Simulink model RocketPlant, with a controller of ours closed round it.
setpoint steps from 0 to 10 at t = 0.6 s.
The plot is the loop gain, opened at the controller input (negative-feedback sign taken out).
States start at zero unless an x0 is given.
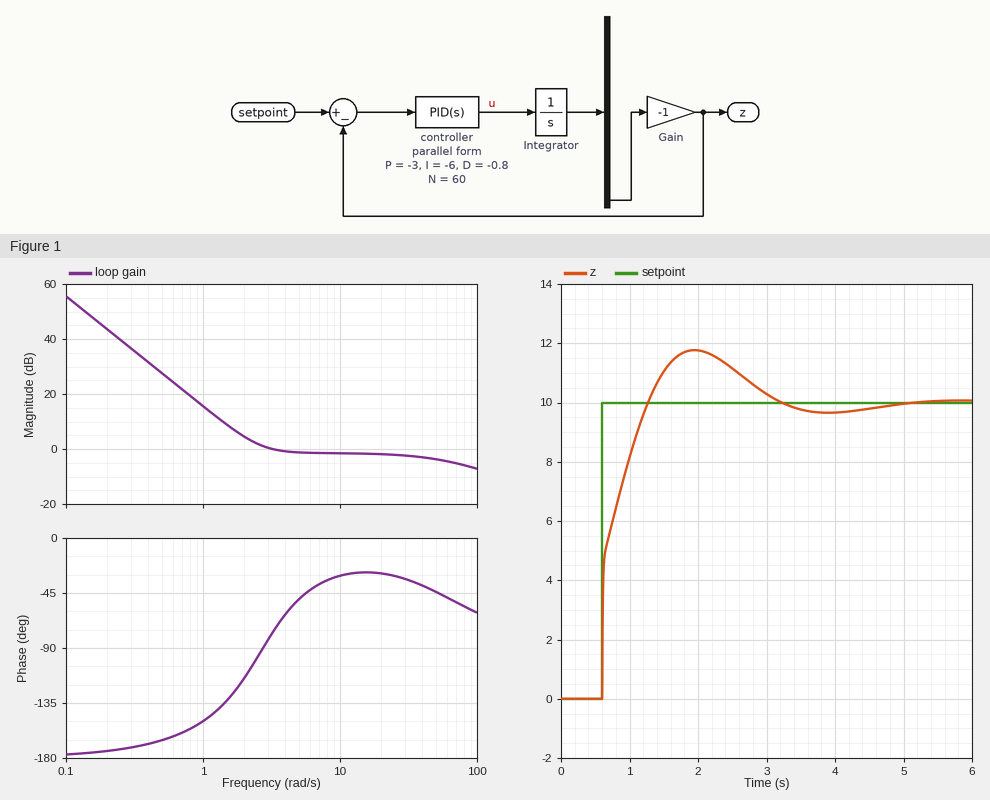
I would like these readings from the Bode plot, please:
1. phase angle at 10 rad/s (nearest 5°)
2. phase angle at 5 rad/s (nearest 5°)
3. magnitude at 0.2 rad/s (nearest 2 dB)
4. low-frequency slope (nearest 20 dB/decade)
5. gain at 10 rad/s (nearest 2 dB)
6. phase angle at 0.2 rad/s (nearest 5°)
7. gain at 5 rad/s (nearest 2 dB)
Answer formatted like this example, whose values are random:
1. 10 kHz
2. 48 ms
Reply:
1. -30°
2. -50°
3. 44 dB
4. -40 dB/decade
5. -2 dB
6. -175°
7. -2 dB
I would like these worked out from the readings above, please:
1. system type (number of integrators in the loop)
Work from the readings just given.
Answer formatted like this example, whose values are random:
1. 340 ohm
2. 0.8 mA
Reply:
1. 2
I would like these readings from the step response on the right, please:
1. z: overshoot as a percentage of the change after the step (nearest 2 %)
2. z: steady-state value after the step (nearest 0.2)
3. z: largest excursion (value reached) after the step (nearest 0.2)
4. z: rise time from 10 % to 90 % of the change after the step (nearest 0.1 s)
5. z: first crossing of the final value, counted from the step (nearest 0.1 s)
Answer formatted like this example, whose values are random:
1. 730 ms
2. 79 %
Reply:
1. 18 %
2. 10.0
3. 11.8
4. 0.5 s
5. 0.7 s
